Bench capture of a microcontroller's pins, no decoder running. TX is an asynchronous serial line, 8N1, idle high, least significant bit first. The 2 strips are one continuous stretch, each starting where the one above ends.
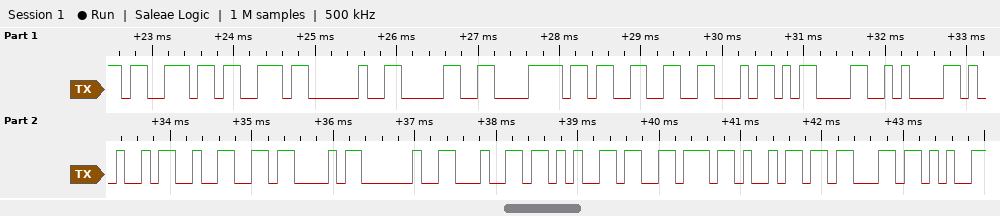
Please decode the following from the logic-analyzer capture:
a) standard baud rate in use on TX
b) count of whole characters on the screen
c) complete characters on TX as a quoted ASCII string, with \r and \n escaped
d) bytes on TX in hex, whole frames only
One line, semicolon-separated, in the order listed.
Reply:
9600 baud; 18; "ss 0x3F\r\nI2C devic"; 73 73 20 30 78 33 46 0D 0A 49 32 43 20 64 65 76 69 63
